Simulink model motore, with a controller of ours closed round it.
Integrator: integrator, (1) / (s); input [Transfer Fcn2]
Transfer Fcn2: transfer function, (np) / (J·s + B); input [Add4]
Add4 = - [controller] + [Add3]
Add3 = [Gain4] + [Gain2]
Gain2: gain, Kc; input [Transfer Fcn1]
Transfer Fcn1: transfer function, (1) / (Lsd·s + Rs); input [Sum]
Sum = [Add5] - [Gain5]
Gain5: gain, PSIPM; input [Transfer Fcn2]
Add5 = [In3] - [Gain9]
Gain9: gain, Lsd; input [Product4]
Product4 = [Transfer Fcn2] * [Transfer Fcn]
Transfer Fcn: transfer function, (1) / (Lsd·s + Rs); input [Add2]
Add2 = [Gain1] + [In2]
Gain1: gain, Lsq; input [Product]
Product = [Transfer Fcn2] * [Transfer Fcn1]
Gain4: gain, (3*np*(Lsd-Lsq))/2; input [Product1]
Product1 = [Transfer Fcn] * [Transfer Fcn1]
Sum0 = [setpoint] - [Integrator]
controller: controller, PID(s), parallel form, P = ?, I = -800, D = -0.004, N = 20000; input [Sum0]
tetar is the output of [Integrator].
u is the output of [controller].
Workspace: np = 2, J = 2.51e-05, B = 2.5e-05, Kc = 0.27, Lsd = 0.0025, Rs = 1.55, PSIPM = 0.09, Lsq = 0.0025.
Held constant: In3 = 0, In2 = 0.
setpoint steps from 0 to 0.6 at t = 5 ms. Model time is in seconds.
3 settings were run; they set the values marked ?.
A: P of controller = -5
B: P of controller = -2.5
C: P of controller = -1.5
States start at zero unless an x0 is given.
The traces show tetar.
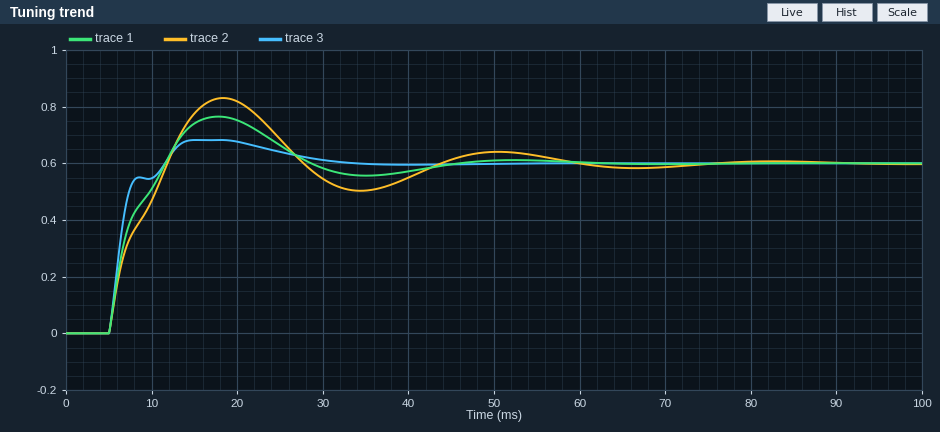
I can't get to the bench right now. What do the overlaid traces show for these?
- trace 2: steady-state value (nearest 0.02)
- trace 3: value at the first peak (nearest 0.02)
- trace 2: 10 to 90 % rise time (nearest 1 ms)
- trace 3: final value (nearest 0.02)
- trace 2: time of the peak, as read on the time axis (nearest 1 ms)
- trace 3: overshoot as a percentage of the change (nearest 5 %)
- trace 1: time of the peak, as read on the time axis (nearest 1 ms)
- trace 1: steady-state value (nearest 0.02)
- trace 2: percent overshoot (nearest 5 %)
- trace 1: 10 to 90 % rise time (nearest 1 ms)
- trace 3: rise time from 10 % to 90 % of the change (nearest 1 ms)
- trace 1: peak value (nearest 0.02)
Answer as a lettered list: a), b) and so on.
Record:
a) 0.60
b) 0.68
c) 6 ms
d) 0.60
e) 18 ms
f) 15 %
g) 18 ms
h) 0.60
i) 40 %
j) 5 ms
k) 3 ms
l) 0.76
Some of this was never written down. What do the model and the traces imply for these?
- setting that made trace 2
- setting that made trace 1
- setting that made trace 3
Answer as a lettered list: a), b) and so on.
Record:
a) C
b) B
c) A
